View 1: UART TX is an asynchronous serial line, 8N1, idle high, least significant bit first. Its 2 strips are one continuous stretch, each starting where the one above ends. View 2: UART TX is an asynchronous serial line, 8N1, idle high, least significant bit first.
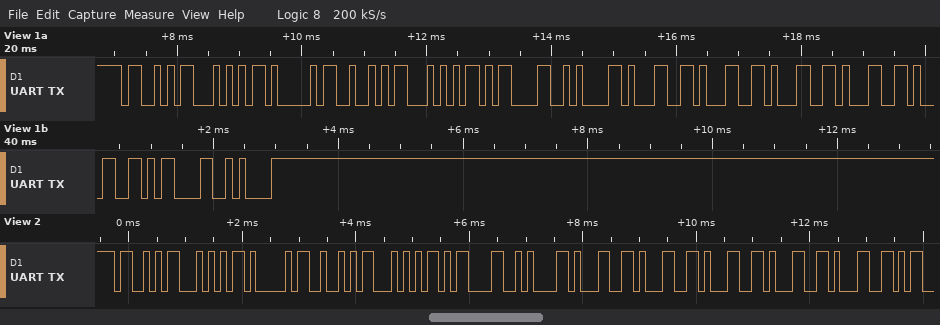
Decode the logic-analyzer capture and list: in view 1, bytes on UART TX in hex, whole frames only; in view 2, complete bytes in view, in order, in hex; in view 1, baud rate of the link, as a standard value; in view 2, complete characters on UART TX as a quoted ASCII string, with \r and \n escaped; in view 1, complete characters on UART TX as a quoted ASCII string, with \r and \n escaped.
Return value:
53 54 41 52 54 0D 0A 31 31 31 31 31 0D 0A
0x53 0x54 0x41 0x52 0x54 0x0D 0x0A 0x31 0x31 0x31 0x31 0x31
9600 baud
"START\r\n11111"
"START\r\n11111\r\n"
